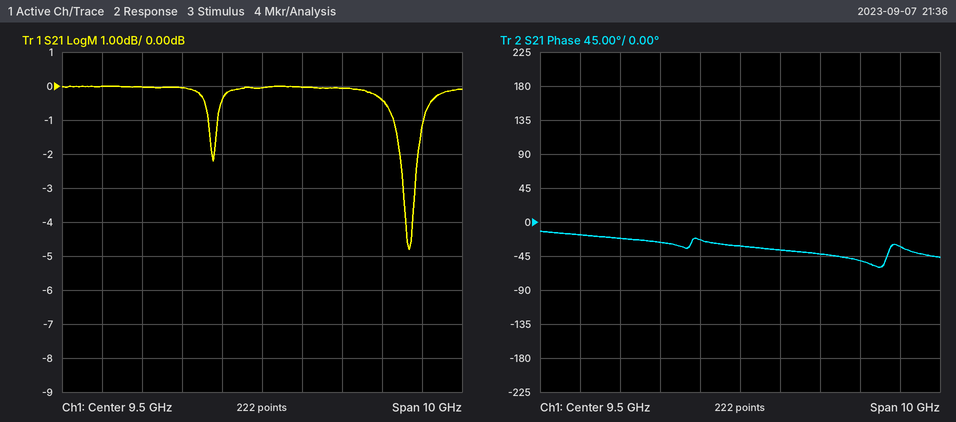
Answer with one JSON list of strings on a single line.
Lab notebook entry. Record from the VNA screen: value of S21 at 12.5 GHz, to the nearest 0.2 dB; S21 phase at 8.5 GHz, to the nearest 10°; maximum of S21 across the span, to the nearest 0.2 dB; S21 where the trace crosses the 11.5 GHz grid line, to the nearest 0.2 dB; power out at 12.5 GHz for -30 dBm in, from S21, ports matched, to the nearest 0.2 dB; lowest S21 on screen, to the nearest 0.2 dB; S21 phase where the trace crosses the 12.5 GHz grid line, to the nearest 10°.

["-0.4 dB", "-20°", "0.0 dB", "0.0 dB", "-30.4 dBm", "-4.8 dB", "-50°"]
